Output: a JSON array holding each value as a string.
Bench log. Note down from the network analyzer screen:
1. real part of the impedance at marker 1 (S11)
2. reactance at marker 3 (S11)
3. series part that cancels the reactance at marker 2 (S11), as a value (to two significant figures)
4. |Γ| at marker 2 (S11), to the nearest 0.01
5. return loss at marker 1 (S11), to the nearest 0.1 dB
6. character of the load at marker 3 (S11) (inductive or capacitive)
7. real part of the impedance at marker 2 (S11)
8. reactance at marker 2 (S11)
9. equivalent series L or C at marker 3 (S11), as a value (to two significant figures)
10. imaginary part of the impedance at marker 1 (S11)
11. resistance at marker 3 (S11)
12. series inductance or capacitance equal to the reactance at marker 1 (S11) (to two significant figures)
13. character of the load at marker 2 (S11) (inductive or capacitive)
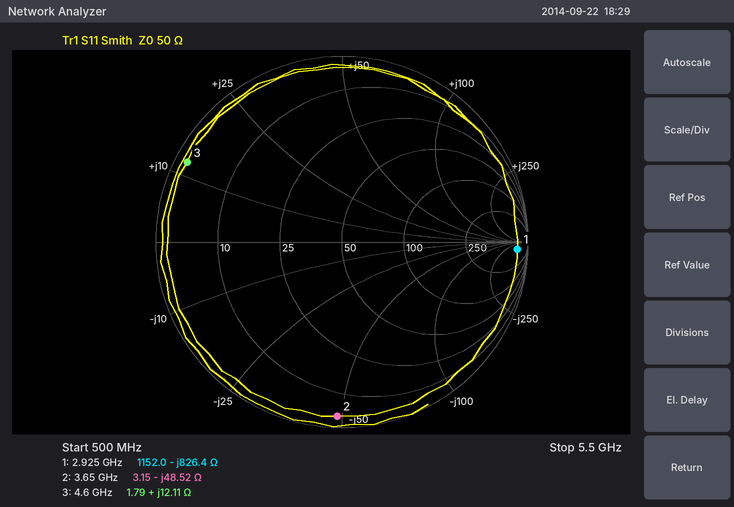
["1152.0 Ω", "+12.11 Ω", "2.1 nH", "0.94", "0.5 dB", "inductive", "3.15 Ω", "-48.52 Ω", "420 pH", "-826.4 Ω", "1.79 Ω", "66 fF", "capacitive"]
